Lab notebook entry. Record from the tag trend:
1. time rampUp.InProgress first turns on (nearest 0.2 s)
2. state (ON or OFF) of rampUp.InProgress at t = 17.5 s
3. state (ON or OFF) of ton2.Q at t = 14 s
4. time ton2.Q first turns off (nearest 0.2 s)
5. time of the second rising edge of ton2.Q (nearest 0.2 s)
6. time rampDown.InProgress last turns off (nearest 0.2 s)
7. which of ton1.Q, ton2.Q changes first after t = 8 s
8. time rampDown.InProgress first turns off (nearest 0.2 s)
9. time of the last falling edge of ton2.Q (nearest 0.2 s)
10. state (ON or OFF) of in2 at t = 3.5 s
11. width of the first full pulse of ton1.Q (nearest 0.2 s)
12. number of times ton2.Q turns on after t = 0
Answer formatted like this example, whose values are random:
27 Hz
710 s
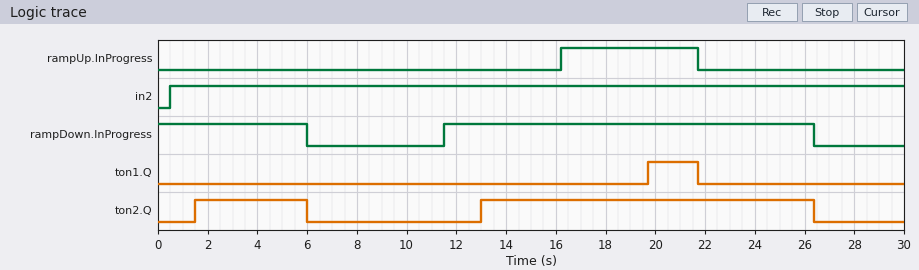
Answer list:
16.2 s
ON
ON
6.0 s
13.0 s
26.4 s
ton2.Q
6.0 s
26.4 s
ON
2.0 s
2
